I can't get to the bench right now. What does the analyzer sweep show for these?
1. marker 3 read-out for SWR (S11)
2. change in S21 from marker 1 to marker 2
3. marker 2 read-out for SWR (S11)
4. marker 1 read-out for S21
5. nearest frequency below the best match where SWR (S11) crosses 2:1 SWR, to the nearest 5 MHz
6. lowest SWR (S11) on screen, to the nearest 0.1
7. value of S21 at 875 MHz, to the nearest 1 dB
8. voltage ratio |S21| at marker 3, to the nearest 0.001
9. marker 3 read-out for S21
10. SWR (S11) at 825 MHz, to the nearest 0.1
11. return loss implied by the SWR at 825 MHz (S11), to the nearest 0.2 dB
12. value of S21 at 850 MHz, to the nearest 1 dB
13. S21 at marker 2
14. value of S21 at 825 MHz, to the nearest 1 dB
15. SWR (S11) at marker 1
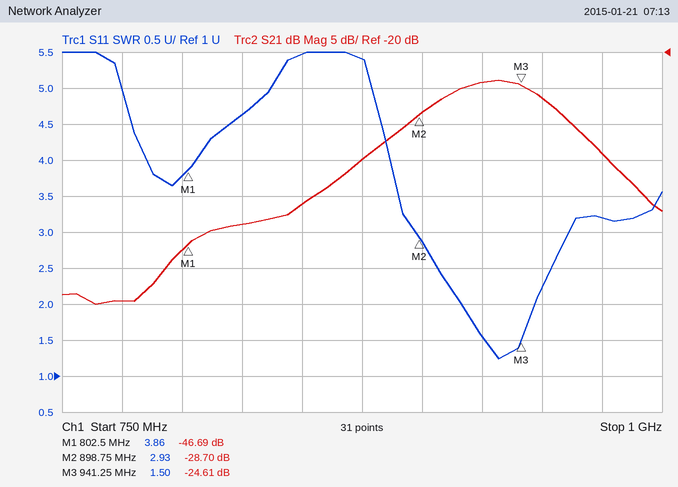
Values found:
1.50
17.99 dB
2.93
-46.69 dB
915 MHz
1.2
-35 dB
0.059
-24.61 dB
4.6
3.8 dB
-41 dB
-28.70 dB
-44 dB
3.86
